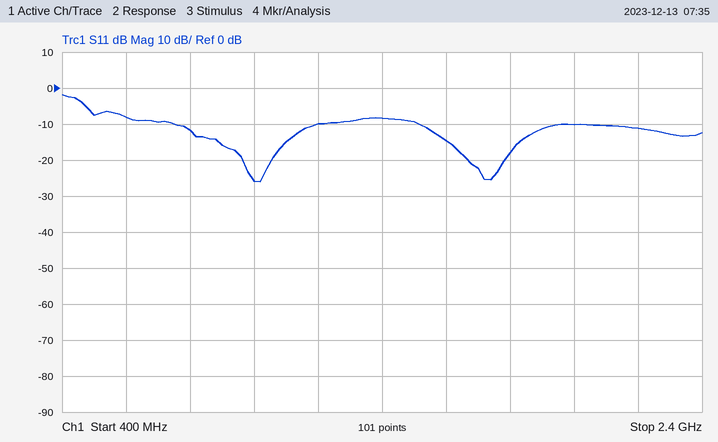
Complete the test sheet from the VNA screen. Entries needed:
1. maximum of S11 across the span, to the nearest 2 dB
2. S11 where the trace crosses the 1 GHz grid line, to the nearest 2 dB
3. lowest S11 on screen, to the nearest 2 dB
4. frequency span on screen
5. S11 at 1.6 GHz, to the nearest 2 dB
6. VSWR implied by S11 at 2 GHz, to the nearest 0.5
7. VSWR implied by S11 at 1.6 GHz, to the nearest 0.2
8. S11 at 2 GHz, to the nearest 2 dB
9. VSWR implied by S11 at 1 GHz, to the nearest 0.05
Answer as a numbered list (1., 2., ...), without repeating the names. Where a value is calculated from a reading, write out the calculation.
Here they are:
1. -2 dB
2. -26 dB
3. -26 dB
4. 2 GHz
5. -14 dB
6. |Γ| = 10^(-10/20) = 0.3162; VSWR = (1 + 0.3162)/(1 − 0.3162) ≈ 1.92, so 2.0 to the nearest 0.5
7. |Γ| = 10^(-14/20) = 0.1995; VSWR = (1 + 0.1995)/(1 − 0.1995) ≈ 1.50, so 1.4 to the nearest 0.2
8. -10 dB
9. |Γ| = 10^(-26/20) = 0.0501; VSWR = (1 + 0.0501)/(1 − 0.0501) ≈ 1.11, so 1.10 to the nearest 0.05
